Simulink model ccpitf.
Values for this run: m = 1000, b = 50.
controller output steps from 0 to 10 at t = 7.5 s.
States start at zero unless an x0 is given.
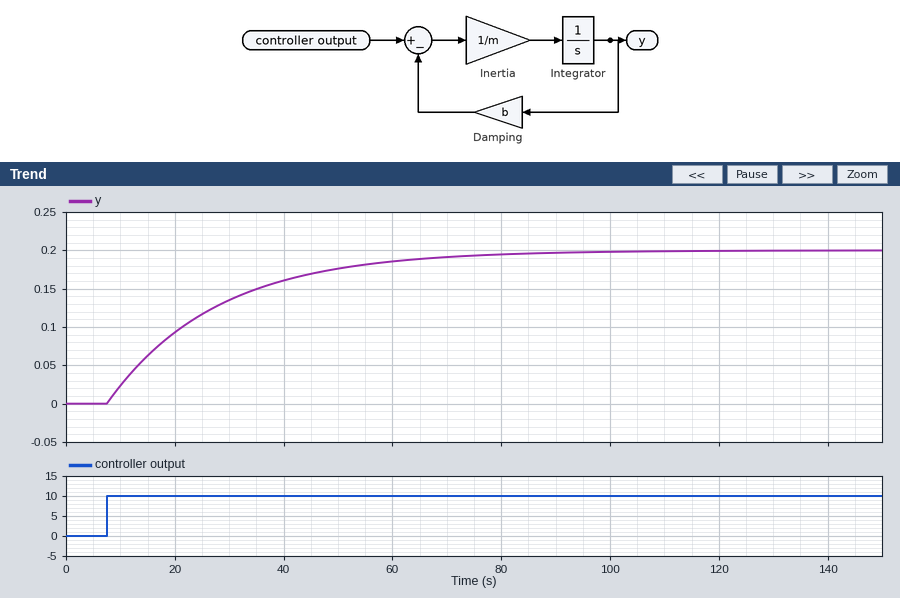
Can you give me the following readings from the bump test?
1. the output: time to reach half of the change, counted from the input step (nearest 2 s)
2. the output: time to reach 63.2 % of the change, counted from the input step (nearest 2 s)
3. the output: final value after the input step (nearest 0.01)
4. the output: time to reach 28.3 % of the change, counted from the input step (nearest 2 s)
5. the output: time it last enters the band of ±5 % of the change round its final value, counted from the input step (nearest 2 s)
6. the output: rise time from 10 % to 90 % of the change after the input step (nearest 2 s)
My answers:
14 s
20 s
0.20
6 s
60 s
44 s
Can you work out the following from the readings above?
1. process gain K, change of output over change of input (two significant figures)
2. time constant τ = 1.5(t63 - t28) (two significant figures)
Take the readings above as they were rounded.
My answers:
0.020
21 s
